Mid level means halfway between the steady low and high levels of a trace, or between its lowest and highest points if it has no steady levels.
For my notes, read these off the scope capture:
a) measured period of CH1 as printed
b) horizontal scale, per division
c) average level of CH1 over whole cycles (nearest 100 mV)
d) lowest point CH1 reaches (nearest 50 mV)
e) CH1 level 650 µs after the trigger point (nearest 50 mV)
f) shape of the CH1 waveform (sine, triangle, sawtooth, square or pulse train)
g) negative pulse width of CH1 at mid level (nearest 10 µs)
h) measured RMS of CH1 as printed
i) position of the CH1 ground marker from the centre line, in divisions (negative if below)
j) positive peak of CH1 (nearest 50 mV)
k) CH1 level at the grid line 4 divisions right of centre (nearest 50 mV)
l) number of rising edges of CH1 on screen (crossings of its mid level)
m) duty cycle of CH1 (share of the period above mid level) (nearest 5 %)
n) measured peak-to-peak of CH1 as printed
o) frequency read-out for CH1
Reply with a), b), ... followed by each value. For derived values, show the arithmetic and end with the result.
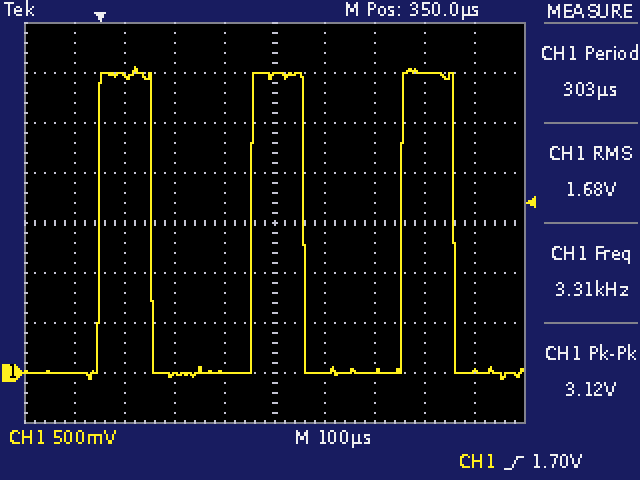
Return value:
a) 303 µs
b) 100 µs
c) -50 mV + 0.35 × (3.05 V − (-50 mV)) ≈ 1.0 V
d) -50 mV
e) 3.00 V
f) pulse train
g) 200 µs
h) 1.68 V
i) -3.0 div
j) 3.05 V
k) 0 mV
l) 3
m) 35 %
n) 3.12 V
o) 3.31 kHz
